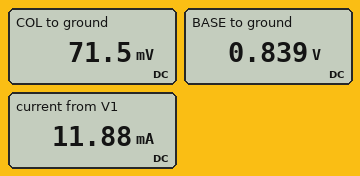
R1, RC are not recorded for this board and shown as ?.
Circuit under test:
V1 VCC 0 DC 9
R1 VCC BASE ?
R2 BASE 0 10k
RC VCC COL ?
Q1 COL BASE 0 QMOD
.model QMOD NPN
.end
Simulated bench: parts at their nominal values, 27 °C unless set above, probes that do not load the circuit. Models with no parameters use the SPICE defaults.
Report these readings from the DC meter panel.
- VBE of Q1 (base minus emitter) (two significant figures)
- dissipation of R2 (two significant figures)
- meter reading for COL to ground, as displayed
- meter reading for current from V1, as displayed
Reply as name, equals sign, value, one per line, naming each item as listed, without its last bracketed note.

VBE of Q1 (base minus emitter) = 840 mV
dissipation of R2 = 70 µW
meter reading for COL to ground, as displayed = 71.5 mV
meter reading for current from V1, as displayed = 11.88 mA
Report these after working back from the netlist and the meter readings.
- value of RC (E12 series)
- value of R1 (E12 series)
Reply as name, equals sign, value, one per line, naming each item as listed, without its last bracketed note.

value of RC = 820 Ω
value of R1 = 8.2 kΩ
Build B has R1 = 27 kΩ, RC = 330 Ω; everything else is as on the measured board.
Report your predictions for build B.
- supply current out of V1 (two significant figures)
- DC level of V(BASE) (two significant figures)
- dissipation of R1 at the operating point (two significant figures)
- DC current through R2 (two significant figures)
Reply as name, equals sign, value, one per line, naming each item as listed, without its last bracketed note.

supply current out of V1 = 22 mA
DC level of V(BASE) = 850 mV
dissipation of R1 at the operating point = 2.5 mW
DC current through R2 = 85 µA
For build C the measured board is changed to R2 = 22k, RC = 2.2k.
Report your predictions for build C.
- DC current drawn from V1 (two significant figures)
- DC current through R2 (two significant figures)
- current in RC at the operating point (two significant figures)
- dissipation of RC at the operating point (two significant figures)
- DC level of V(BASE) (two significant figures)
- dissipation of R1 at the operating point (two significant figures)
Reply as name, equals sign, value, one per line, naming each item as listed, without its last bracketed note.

DC current drawn from V1 = 5.1 mA
DC current through R2 = 37 µA
current in RC at the operating point = 4.1 mA
dissipation of RC at the operating point = 36 mW
DC level of V(BASE) = 820 mV
dissipation of R1 at the operating point = 8.2 mW
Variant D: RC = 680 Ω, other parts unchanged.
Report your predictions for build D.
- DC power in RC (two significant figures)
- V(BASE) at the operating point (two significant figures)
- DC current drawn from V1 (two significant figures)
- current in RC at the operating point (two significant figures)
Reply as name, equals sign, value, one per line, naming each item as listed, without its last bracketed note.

DC power in RC = 120 mW
V(BASE) at the operating point = 840 mV
DC current drawn from V1 = 14 mA
current in RC at the operating point = 13 mA
